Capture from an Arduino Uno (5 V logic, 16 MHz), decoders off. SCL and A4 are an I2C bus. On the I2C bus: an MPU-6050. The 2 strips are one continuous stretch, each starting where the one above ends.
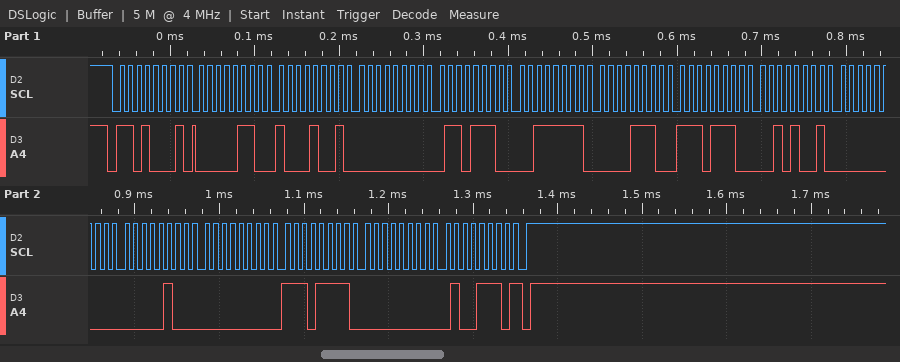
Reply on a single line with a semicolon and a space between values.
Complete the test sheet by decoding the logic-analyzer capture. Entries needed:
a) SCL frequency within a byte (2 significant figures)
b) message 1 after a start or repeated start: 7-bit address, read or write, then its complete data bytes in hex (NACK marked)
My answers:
100 kHz; 0x68 read: 06 89 00 6E 3F 0E EE 29 00 04 00 EF 00 4E NACK
